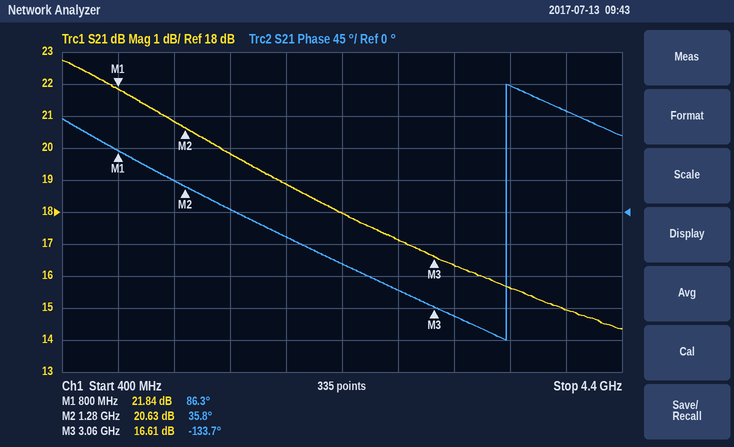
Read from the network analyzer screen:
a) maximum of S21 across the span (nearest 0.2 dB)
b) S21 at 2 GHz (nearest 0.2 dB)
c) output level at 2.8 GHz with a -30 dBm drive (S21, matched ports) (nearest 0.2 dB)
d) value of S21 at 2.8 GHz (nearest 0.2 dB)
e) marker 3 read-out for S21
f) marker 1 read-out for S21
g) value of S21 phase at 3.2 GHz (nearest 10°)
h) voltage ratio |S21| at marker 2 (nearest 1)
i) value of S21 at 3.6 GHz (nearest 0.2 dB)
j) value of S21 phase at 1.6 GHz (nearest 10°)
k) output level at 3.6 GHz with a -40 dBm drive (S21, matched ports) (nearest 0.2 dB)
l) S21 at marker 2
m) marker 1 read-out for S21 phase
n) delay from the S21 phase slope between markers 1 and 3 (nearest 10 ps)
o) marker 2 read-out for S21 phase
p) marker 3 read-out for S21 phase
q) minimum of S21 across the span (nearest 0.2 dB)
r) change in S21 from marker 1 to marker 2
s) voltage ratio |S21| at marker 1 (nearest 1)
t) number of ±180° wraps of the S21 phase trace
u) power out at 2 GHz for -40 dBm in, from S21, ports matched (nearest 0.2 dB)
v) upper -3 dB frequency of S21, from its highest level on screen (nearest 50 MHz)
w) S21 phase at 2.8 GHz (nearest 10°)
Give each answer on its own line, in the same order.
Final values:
22.8 dB
18.8 dB
-12.8 dBm
17.2 dB
16.61 dB
21.84 dB
-150°
11
15.6 dB
0°
-24.4 dBm
20.63 dB
86.3°
270 ps
35.8°
-133.7°
14.4 dB
-1.21 dB
12
1
-21.2 dBm
1.65 GHz
-110°
